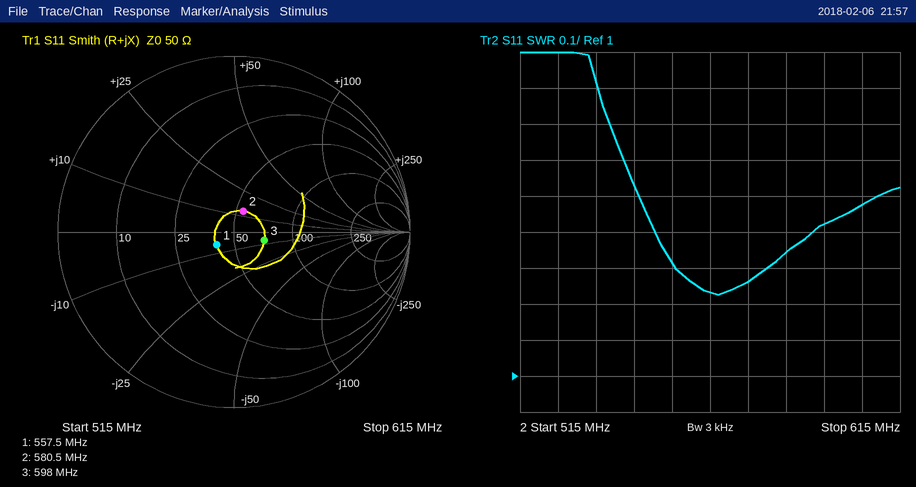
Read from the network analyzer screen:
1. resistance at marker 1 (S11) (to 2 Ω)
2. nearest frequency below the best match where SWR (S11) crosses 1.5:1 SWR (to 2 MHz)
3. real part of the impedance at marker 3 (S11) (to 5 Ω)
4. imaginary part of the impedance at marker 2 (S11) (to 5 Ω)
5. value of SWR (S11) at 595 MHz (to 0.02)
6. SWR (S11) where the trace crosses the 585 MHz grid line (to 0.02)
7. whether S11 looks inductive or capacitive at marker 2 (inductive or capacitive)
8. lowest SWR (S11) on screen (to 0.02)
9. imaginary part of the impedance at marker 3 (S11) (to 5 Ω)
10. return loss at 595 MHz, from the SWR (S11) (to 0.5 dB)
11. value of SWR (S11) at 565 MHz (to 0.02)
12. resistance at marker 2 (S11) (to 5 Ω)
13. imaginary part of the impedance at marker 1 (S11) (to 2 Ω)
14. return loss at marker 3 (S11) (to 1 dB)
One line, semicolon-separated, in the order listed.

40 Ω; 546 MHz; 70 Ω; +15 Ω; 1.42; 1.34; inductive; 1.22; -5 Ω; 15.0 dB; 1.24; 55 Ω; -6 Ω; 15 dB
